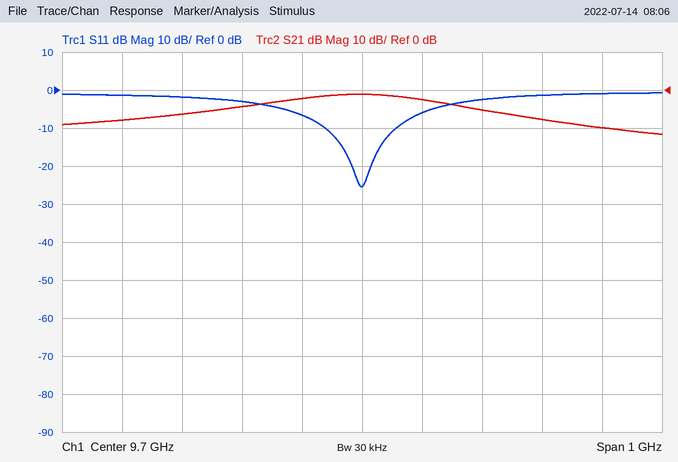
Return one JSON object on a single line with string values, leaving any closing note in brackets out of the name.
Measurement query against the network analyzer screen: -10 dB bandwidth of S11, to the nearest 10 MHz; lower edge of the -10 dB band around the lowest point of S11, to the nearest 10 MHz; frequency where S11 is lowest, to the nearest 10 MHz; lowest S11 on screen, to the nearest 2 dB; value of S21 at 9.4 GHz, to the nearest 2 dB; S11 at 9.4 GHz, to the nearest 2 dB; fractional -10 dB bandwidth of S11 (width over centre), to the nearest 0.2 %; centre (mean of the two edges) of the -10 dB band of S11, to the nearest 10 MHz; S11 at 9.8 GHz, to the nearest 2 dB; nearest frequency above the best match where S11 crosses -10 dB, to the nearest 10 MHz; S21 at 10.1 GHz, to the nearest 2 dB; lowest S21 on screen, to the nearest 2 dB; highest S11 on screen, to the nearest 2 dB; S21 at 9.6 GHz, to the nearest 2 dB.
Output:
{"-10 dB bandwidth of S11, to the nearest 10 MHz": "120 MHz", "lower edge of the -10 dB band around the lowest point of S11, to the nearest 10 MHz": "9.64 GHz", "frequency where S11 is lowest, to the nearest 10 MHz": "9.70 GHz", "lowest S11 on screen, to the nearest 2 dB": "-26 dB", "value of S21 at 9.4 GHz, to the nearest 2 dB": "-6 dB", "S11 at 9.4 GHz, to the nearest 2 dB": "-2 dB", "fractional -10 dB bandwidth of S11 (width over centre), to the nearest 0.2 %": "1.2 %", "centre (mean of the two edges) of the -10 dB band of S11, to the nearest 10 MHz": "9.70 GHz", "S11 at 9.8 GHz, to the nearest 2 dB": "-6 dB", "nearest frequency above the best match where S11 crosses -10 dB, to the nearest 10 MHz": "9.76 GHz", "S21 at 10.1 GHz, to the nearest 2 dB": "-10 dB", "lowest S21 on screen, to the nearest 2 dB": "-12 dB", "highest S11 on screen, to the nearest 2 dB": "0 dB", "S21 at 9.6 GHz, to the nearest 2 dB": "-2 dB"}
